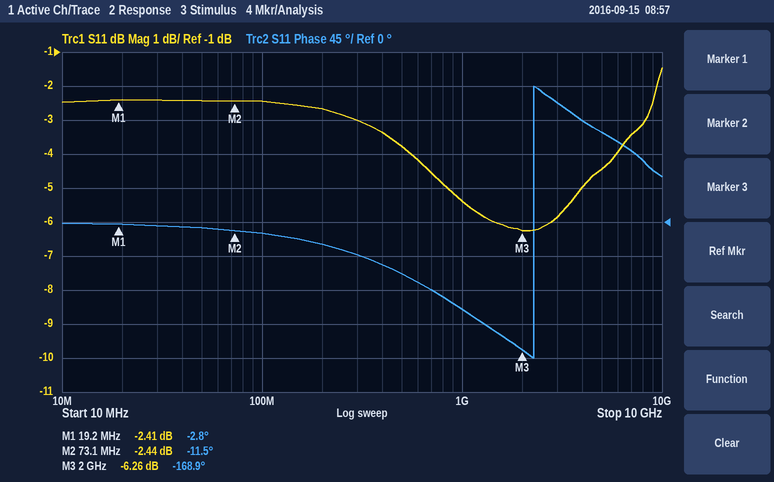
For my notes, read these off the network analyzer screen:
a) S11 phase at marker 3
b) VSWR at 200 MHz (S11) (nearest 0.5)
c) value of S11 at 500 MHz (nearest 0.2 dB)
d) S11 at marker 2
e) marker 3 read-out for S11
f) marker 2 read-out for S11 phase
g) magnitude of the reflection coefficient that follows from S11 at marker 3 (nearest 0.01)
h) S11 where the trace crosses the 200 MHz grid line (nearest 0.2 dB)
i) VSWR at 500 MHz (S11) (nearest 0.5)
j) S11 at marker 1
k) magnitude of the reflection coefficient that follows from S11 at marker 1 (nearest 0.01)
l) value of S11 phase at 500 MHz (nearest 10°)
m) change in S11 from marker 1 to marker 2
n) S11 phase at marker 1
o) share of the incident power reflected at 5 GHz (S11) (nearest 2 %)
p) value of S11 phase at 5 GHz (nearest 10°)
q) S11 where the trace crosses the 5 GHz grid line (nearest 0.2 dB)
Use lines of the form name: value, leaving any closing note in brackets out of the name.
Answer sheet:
S11 phase at marker 3: -168.9°
VSWR at 200 MHz (S11): 6.5
value of S11 at 500 MHz: -3.8 dB
S11 at marker 2: -2.44 dB
marker 3 read-out for S11: -6.26 dB
marker 2 read-out for S11 phase: -11.5°
magnitude of the reflection coefficient that follows from S11 at marker 3: 0.49
S11 where the trace crosses the 200 MHz grid line: -2.6 dB
VSWR at 500 MHz (S11): 4.5
S11 at marker 1: -2.41 dB
magnitude of the reflection coefficient that follows from S11 at marker 1: 0.76
value of S11 phase at 500 MHz: -70°
change in S11 from marker 1 to marker 2: -0.03 dB
S11 phase at marker 1: -2.8°
share of the incident power reflected at 5 GHz (S11): 36 %
value of S11 phase at 5 GHz: 120°
S11 where the trace crosses the 5 GHz grid line: -4.4 dB
